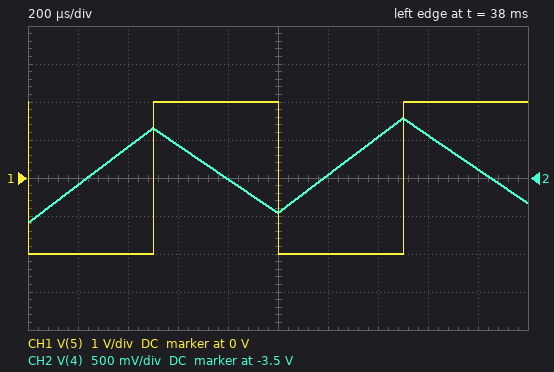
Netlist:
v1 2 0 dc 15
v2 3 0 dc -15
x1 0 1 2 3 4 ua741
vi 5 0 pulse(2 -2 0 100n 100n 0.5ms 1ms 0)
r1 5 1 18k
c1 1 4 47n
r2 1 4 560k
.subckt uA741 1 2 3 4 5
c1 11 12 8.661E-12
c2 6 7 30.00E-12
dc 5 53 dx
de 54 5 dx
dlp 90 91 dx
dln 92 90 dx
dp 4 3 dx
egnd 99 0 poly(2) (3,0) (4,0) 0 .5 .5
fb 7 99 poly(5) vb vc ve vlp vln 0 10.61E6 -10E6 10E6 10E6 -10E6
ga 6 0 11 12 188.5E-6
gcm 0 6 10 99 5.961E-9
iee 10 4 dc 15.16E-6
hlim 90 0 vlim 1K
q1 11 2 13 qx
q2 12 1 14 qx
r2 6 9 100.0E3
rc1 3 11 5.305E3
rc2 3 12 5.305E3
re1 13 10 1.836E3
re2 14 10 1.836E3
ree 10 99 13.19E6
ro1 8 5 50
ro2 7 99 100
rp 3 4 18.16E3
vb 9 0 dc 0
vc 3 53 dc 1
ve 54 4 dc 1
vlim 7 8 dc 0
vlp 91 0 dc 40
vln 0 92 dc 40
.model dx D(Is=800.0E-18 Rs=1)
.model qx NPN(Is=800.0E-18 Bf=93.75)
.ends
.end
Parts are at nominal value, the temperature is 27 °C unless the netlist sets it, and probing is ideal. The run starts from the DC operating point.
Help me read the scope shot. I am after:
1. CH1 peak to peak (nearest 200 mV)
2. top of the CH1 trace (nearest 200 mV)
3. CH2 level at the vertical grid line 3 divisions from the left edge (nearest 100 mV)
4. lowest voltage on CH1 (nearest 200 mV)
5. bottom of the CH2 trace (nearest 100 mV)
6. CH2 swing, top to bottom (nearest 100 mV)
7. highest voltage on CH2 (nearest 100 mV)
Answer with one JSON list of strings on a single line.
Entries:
["4.0 V", "2.0 V", "-3.1 V", "-2.0 V", "-4.1 V", "1.4 V", "-2.7 V"]
